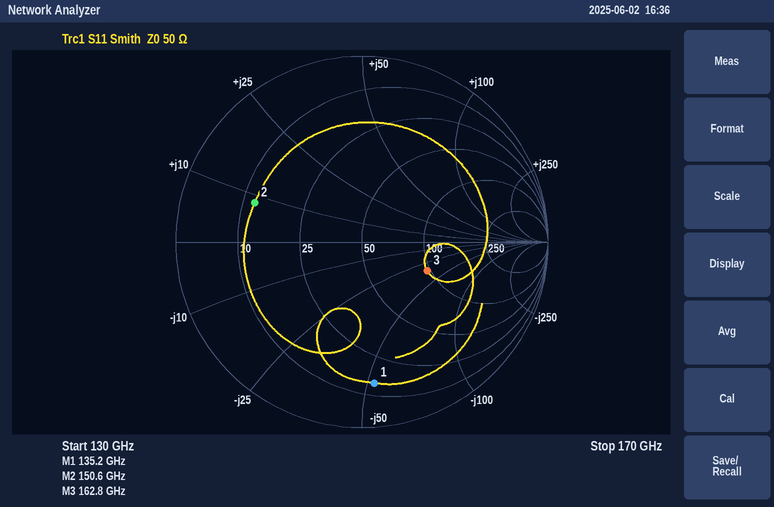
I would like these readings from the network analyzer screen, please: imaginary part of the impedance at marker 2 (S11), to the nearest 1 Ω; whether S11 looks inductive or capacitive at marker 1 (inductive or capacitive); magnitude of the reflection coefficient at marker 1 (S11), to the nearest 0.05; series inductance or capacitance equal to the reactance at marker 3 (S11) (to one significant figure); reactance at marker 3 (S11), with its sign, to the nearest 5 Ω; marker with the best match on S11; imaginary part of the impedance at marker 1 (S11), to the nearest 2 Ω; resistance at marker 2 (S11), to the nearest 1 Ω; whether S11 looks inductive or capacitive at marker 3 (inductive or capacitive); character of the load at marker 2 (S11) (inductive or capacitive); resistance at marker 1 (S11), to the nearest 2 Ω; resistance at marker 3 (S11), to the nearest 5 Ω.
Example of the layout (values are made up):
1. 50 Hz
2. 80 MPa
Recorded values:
1. +8 Ω
2. capacitive
3. 0.75
4. 30 fF
5. -35 Ω
6. marker 3
7. -52 Ω
8. 12 Ω
9. capacitive
10. inductive
11. 14 Ω
12. 95 Ω
